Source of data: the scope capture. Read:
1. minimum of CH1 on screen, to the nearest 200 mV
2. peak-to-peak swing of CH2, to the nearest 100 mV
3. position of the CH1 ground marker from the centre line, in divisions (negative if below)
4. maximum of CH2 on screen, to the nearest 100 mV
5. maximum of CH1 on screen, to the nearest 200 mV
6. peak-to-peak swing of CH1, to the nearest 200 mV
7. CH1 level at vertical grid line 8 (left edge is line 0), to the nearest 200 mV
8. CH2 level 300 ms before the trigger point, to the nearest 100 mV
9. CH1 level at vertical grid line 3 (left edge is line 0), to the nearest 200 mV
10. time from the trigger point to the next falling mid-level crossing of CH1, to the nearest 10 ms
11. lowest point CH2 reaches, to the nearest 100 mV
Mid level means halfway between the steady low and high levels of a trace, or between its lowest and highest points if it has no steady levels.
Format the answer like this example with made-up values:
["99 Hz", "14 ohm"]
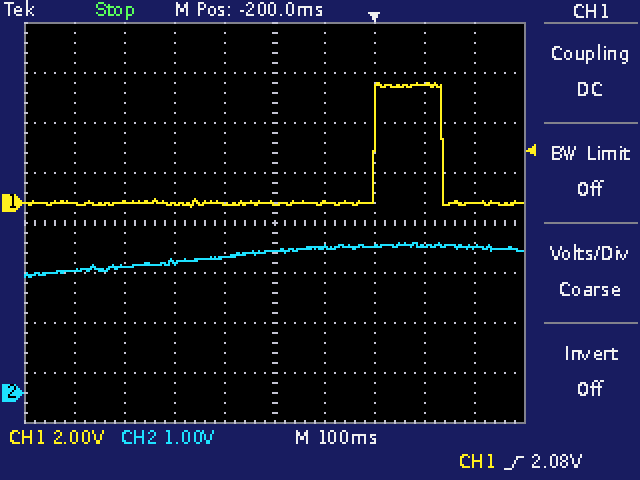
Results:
["-200 mV", "700 mV", "+0.4 div", "3.0 V", "4.8 V", "5.0 V", "4.8 V", "2.7 V", "0.0 V", "140 ms", "2.3 V"]
